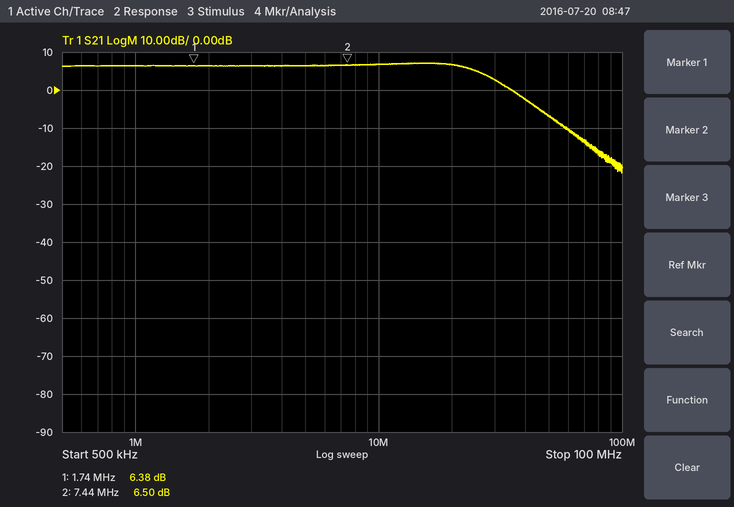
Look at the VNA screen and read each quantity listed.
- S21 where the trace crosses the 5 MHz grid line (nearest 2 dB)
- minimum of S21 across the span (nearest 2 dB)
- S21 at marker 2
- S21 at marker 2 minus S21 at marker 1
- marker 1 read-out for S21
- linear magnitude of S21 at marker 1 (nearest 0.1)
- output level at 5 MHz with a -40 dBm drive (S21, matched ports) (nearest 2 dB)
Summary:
6 dB
-22 dB
6.50 dB
0.12 dB
6.38 dB
2.1
-34 dBm
